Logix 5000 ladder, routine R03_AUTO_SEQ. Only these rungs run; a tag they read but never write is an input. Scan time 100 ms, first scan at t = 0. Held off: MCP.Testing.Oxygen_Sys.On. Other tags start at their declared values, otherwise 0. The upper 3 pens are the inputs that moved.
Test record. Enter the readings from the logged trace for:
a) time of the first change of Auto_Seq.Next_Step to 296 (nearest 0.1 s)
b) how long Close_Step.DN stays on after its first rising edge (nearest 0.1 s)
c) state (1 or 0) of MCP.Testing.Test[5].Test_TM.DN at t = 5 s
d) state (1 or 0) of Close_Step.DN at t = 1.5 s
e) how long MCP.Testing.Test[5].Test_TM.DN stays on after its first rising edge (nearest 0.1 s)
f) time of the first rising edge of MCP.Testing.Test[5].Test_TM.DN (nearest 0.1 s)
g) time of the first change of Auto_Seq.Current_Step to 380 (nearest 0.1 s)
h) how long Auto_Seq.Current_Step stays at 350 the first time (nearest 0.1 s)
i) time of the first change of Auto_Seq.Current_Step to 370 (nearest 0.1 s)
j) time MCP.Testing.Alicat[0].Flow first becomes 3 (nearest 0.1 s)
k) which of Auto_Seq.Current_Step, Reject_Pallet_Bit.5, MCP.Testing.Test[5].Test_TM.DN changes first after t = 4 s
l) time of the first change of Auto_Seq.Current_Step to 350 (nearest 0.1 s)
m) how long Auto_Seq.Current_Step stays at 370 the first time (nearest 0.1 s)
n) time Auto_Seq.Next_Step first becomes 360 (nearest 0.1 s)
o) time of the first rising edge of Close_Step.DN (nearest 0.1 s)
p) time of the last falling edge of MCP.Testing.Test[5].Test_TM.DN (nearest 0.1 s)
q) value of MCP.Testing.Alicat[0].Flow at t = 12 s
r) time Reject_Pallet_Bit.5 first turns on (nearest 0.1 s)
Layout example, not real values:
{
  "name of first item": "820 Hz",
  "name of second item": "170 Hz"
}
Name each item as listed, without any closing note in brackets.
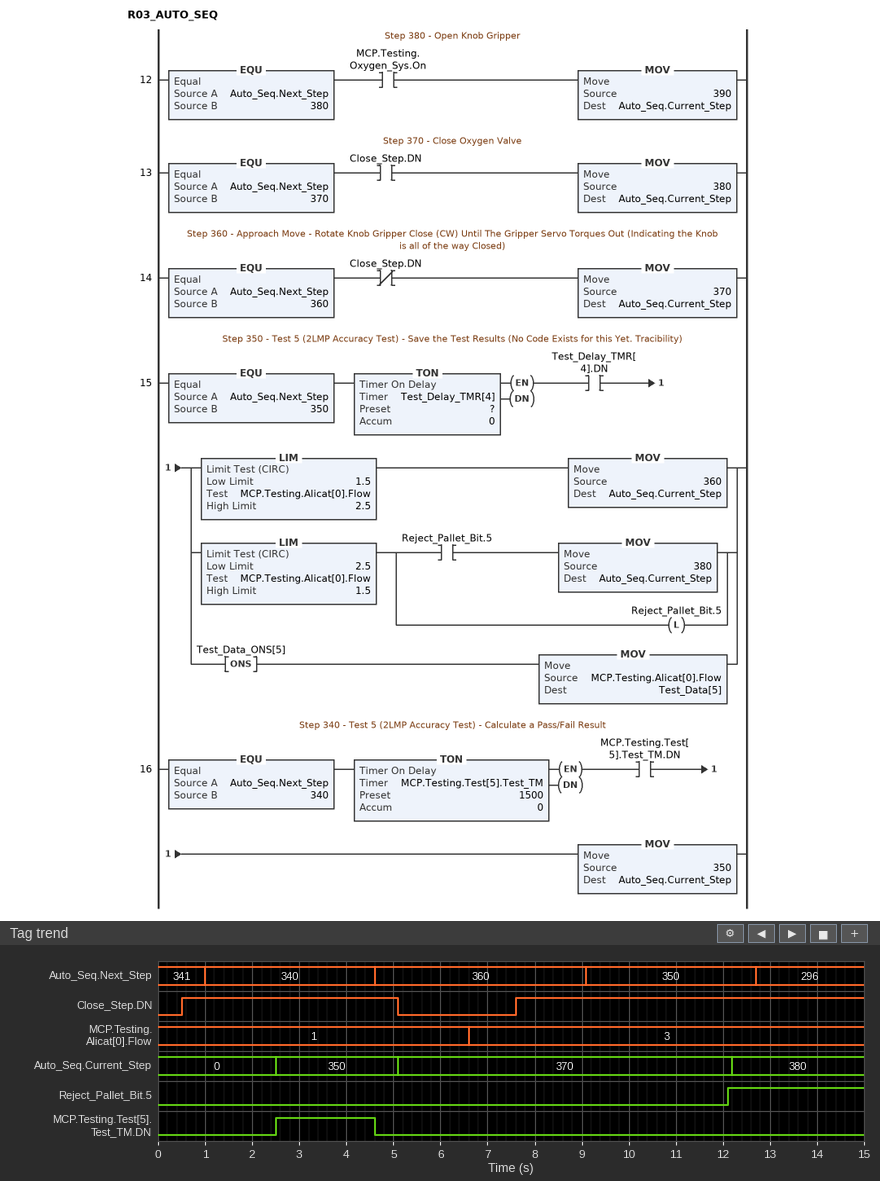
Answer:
{
  "time of the first change of Auto_Seq.Next_Step to 296": "12.7 s",
  "how long Close_Step.DN stays on after its first rising edge": "4.6 s",
  "state (1 or 0) of MCP.Testing.Test[5].Test_TM.DN at t = 5 s": "0",
  "state (1 or 0) of Close_Step.DN at t = 1.5 s": "1",
  "how long MCP.Testing.Test[5].Test_TM.DN stays on after its first rising edge": "2.1 s",
  "time of the first rising edge of MCP.Testing.Test[5].Test_TM.DN": "2.5 s",
  "time of the first change of Auto_Seq.Current_Step to 380": "12.2 s",
  "how long Auto_Seq.Current_Step stays at 350 the first time": "2.6 s",
  "time of the first change of Auto_Seq.Current_Step to 370": "5.1 s",
  "time MCP.Testing.Alicat[0].Flow first becomes 3": "6.6 s",
  "which of Auto_Seq.Current_Step, Reject_Pallet_Bit.5, MCP.Testing.Test[5].Test_TM.DN changes first after t = 4 s": "MCP.Testing.Test[5].Test_TM.DN",
  "time of the first change of Auto_Seq.Current_Step to 350": "2.5 s",
  "how long Auto_Seq.Current_Step stays at 370 the first time": "7.1 s",
  "time Auto_Seq.Next_Step first becomes 360": "4.6 s",
  "time of the first rising edge of Close_Step.DN": "0.5 s",
  "time of the last falling edge of MCP.Testing.Test[5].Test_TM.DN": "4.6 s",
  "value of MCP.Testing.Alicat[0].Flow at t = 12 s": "3",
  "time Reject_Pallet_Bit.5 first turns on": "12.1 s"
}
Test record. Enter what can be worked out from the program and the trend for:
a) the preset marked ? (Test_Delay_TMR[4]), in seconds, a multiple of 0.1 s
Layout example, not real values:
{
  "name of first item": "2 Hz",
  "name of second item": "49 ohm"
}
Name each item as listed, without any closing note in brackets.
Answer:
{
  "the preset marked ? (Test_Delay_TMR[4]), in seconds, a multiple of 0.1 s": "3.0 s"
}
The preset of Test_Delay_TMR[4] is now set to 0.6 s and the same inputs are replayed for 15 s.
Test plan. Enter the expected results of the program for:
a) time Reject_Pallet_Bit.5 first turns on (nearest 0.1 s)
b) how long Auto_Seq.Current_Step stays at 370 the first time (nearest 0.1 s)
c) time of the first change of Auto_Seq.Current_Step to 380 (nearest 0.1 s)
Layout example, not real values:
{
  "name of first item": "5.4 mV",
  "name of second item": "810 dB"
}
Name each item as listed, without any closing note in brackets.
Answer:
{
  "time Reject_Pallet_Bit.5 first turns on": "9.7 s",
  "how long Auto_Seq.Current_Step stays at 370 the first time": "4.7 s",
  "time of the first change of Auto_Seq.Current_Step to 380": "9.8 s"
}
